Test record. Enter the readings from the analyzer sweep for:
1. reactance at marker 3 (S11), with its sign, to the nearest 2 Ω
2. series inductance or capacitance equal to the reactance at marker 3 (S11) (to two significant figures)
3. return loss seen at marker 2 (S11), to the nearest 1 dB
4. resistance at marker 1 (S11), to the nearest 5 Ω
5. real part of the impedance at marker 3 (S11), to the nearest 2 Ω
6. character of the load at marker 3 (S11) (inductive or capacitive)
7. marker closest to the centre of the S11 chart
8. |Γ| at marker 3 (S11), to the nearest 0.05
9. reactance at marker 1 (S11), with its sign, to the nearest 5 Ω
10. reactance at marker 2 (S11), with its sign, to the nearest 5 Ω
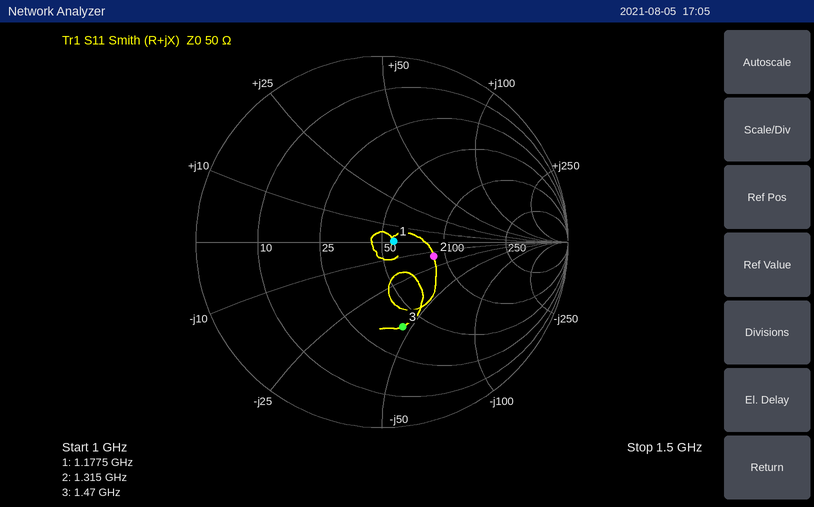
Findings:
-46 Ω
2.4 pF
11 dB
55 Ω
40 Ω
capacitive
marker 1
0.45
0 Ω
-15 Ω
